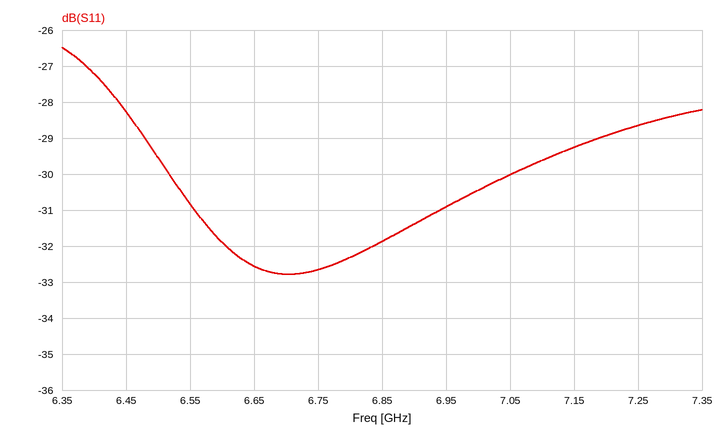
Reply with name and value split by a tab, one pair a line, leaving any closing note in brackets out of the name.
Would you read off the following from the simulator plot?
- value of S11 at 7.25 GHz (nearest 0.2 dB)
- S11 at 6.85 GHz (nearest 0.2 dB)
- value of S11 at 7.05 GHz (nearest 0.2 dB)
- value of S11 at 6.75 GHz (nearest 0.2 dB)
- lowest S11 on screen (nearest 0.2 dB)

value of S11 at 7.25 GHz	-28.6 dB
S11 at 6.85 GHz	-31.8 dB
value of S11 at 7.05 GHz	-30.0 dB
value of S11 at 6.75 GHz	-32.6 dB
lowest S11 on screen	-32.8 dB
